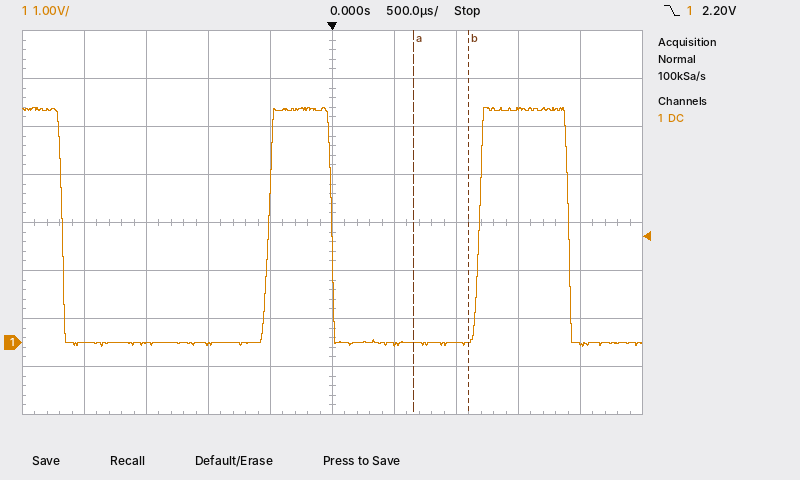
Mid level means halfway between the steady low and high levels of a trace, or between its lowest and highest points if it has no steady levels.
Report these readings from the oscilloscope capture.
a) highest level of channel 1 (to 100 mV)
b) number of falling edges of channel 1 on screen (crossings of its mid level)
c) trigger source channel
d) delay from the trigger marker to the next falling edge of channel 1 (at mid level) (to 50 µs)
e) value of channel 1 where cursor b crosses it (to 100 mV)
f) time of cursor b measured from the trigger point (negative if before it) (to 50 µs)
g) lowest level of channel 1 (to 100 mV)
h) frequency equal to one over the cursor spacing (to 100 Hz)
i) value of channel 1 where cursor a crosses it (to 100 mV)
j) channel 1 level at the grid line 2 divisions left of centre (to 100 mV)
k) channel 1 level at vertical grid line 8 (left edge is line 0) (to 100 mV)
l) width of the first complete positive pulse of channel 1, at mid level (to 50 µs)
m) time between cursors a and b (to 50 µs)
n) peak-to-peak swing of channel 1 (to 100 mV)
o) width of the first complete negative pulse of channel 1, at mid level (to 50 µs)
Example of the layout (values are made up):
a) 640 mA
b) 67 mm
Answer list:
a) 4.9 V
b) 3
c) channel 1
d) 1.90 ms
e) 0.0 V
f) +1.10 ms
g) -100 mV
h) 2.2 kHz
i) 0.0 V
j) 0.0 V
k) 4.9 V
l) 500 µs
m) 450 µs
n) 5.0 V
o) 1.65 ms
